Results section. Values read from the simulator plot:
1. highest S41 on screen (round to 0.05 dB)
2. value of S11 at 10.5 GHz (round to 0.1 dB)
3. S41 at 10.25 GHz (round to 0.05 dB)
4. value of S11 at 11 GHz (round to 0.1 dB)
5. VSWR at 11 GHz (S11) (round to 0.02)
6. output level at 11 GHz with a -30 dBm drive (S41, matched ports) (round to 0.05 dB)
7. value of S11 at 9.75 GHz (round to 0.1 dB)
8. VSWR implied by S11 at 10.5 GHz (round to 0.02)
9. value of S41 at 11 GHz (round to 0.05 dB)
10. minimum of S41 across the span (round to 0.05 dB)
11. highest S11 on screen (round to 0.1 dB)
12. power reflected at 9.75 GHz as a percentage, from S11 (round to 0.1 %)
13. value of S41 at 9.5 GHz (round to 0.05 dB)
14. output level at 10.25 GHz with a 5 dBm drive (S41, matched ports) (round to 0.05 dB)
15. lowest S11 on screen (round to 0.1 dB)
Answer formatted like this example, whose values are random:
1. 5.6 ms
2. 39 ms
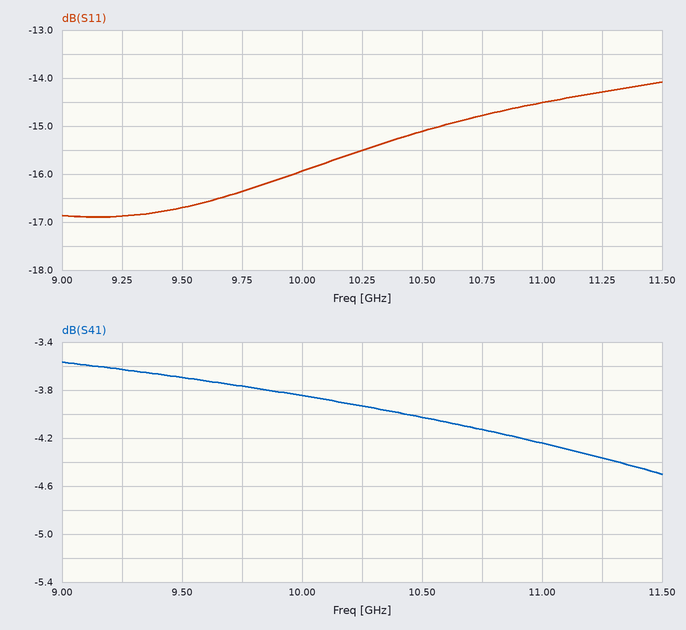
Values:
1. -3.55 dB
2. -15.1 dB
3. -3.95 dB
4. -14.5 dB
5. 1.46
6. -34.25 dBm
7. -16.4 dB
8. 1.42
9. -4.25 dB
10. -4.50 dB
11. -14.1 dB
12. 2.3 %
13. -3.70 dB
14. 1.05 dBm
15. -16.9 dB
